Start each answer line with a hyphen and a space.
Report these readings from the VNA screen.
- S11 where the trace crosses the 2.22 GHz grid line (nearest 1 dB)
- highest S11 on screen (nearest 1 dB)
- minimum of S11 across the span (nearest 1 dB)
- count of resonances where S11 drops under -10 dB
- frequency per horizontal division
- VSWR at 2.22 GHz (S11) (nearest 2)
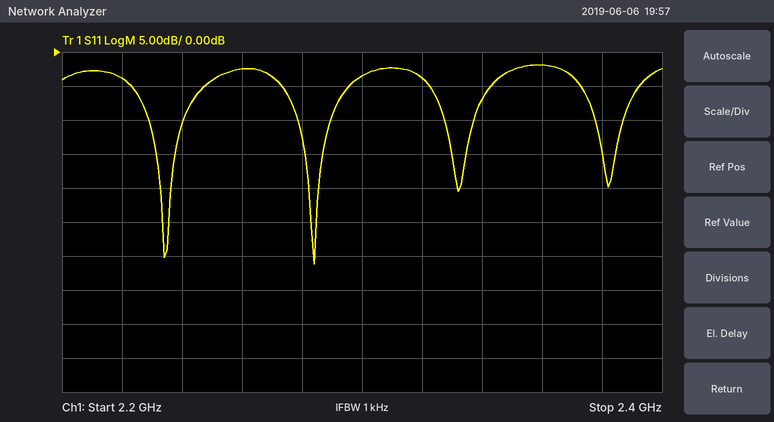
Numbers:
- -4 dB
- -2 dB
- -31 dB
- 4
- 20 MHz
- 4
